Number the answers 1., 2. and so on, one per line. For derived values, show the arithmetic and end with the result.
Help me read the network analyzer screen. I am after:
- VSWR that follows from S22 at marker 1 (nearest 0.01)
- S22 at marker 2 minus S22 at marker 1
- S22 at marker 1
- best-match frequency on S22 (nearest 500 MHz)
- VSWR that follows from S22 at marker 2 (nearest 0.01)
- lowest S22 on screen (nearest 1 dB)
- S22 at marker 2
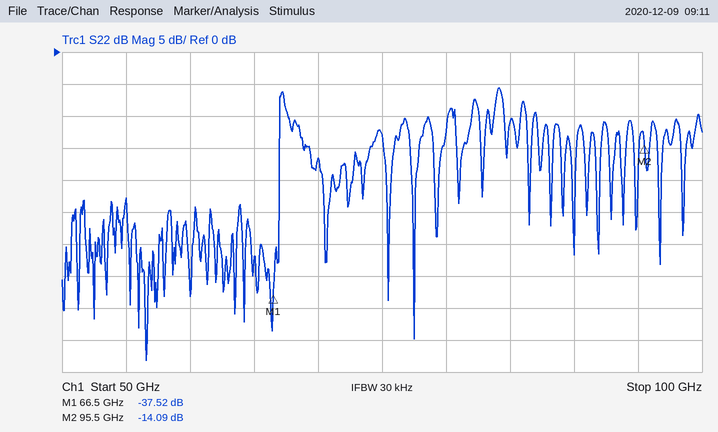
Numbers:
1. (1 + 0.0133)/(1 − 0.0133) ≈ 1.03
2. -14.09 − (-37.52) = 23.43 dB
3. -37.52 dB
4. 56.5 GHz
5. (1 + 0.1975)/(1 − 0.1975) ≈ 1.49
6. -48 dB
7. -14.09 dB
